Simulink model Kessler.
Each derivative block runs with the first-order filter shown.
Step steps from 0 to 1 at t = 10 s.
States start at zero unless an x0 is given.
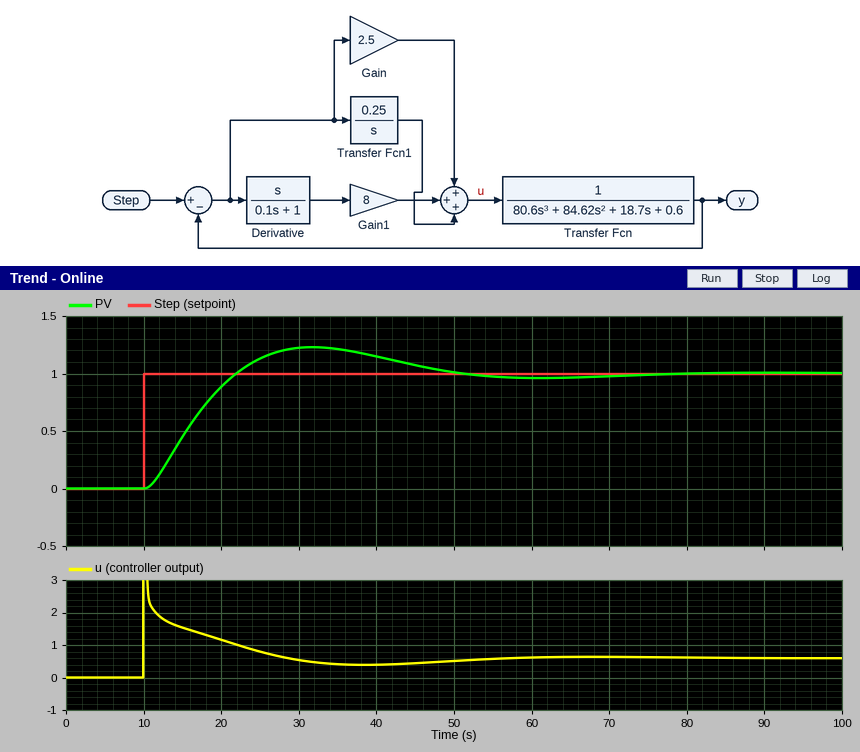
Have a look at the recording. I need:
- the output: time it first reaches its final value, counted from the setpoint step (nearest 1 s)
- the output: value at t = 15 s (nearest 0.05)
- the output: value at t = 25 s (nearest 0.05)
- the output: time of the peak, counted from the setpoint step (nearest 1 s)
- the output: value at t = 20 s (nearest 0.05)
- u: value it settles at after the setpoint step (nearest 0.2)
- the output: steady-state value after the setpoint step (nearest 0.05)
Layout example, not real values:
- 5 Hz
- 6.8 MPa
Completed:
- 12 s
- 0.45
- 1.15
- 22 s
- 0.90
- 0.6
- 1.00
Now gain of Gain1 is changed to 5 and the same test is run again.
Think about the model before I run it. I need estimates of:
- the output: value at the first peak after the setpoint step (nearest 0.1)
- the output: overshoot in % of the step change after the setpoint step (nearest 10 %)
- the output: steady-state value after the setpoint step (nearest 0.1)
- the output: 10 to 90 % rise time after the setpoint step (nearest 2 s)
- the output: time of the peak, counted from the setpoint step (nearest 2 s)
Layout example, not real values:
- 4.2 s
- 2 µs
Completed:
- 1.3
- 30 %
- 1.0
- 8 s
- 20 s
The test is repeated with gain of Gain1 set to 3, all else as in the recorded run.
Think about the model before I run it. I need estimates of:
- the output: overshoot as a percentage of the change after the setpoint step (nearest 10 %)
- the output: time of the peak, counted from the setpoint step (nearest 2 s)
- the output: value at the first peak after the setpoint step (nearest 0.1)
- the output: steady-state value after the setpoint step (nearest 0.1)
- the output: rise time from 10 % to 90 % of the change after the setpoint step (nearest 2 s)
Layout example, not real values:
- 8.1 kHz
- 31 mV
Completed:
- 40 %
- 20 s
- 1.4
- 1.0
- 8 s
